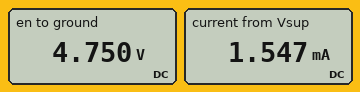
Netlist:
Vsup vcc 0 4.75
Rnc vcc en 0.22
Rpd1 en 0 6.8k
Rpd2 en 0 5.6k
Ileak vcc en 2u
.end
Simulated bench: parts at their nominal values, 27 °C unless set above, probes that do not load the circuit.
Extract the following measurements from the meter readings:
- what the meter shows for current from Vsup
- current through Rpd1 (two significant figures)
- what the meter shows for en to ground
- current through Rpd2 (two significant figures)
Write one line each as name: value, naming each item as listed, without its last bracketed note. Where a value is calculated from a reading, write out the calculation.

what the meter shows for current from Vsup: 1.547 mA
current through Rpd1: (4.75 V) / 6.8 kΩ = 700 µA
what the meter shows for en to ground: 4.750 V
current through Rpd2: (4.75 V) / 5.6 kΩ = 850 µA
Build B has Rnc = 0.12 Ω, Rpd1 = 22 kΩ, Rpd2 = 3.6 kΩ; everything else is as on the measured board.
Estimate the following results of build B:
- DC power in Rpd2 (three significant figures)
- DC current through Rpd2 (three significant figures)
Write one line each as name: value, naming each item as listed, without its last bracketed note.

DC power in Rpd2: 6.27 mW
DC current through Rpd2: 1.32 mA
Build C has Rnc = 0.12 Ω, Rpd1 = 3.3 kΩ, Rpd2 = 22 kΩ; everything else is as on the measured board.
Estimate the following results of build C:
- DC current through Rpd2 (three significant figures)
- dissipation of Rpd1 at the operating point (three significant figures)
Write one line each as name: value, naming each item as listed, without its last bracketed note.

DC current through Rpd2: 216 µA
dissipation of Rpd1 at the operating point: 6.84 mW
